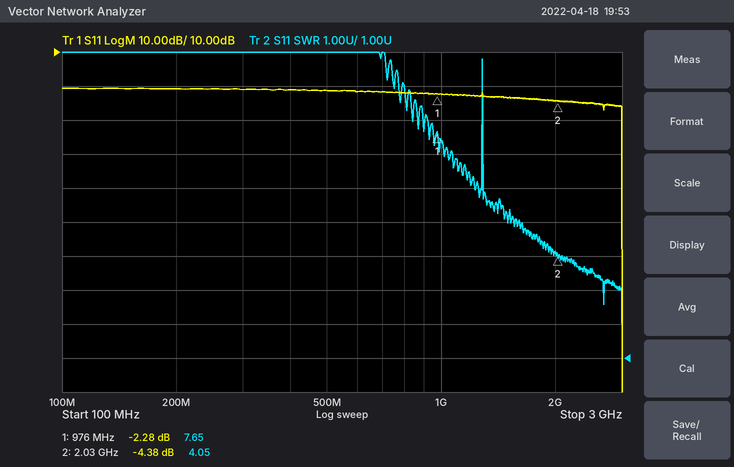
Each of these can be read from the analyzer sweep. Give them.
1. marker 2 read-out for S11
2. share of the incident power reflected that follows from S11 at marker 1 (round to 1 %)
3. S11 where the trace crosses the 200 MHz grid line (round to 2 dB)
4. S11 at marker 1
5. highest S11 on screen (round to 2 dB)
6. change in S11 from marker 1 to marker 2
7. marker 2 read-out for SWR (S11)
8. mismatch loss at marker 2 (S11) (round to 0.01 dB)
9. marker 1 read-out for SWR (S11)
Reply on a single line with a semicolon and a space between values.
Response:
-4.38 dB; 59 %; 0 dB; -2.28 dB; 0 dB; -2.10 dB; 4.05; 1.97 dB; 7.65
